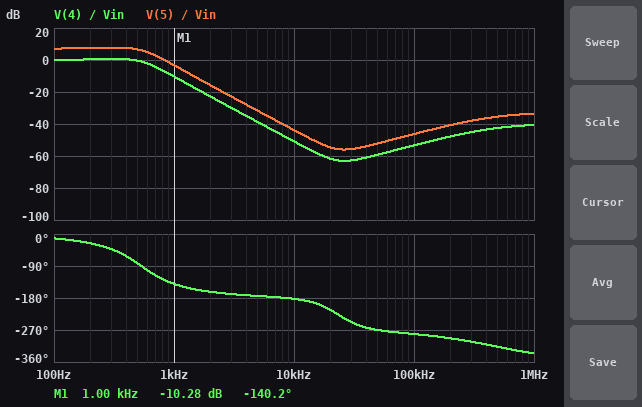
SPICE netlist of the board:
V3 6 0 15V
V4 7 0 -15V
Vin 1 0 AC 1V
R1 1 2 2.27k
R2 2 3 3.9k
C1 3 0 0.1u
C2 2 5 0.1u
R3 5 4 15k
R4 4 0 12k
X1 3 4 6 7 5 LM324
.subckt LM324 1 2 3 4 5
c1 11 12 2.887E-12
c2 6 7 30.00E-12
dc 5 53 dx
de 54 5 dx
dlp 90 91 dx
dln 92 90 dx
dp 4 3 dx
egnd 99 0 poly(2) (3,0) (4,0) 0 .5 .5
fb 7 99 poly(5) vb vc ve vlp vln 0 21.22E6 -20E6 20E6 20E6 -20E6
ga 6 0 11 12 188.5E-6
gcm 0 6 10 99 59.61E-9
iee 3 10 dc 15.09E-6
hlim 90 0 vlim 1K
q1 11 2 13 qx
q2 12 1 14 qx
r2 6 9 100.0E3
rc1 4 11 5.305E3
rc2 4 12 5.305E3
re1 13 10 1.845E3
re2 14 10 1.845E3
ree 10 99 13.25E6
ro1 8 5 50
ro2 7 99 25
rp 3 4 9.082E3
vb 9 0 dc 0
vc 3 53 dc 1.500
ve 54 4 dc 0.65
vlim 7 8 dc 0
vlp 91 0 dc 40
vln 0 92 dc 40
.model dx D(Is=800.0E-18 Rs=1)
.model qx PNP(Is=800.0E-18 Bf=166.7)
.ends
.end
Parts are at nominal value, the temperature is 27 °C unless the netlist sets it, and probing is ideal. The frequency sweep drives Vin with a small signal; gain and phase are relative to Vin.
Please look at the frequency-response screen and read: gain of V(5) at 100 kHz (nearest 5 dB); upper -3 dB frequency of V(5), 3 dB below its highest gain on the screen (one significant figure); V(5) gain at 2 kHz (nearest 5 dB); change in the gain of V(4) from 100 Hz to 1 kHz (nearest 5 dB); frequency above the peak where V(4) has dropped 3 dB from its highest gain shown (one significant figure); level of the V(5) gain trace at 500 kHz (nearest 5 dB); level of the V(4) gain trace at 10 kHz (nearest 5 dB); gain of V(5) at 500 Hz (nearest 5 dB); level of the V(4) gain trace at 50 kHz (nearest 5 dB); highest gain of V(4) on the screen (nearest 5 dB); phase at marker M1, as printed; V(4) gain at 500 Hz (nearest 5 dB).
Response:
-45 dB
600 Hz
-15 dB
-10 dB
600 Hz
-35 dB
-50 dB
5 dB
-60 dB
0 dB
-140.2 deg
0 dB
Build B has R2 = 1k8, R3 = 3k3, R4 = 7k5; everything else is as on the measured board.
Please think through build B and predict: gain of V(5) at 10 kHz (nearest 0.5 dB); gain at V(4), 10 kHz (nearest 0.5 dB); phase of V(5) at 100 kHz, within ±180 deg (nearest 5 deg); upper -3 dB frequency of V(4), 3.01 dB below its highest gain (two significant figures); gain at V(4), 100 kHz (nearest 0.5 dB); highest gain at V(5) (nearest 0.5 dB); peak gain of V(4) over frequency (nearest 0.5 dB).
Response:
-41.0 dB
-44.0 dB
85 deg
730 Hz
-53.0 dB
3.0 dB
0 dB
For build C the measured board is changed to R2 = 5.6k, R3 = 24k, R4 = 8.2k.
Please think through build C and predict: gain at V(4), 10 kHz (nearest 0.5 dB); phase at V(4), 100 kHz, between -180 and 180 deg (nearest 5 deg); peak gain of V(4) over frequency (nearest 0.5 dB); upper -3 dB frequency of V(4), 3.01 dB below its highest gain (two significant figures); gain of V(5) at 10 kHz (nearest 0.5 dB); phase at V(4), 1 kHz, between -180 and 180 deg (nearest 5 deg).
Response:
-54.0 dB
70 deg
9.5 dB
500 Hz
-42.0 dB
-170 deg
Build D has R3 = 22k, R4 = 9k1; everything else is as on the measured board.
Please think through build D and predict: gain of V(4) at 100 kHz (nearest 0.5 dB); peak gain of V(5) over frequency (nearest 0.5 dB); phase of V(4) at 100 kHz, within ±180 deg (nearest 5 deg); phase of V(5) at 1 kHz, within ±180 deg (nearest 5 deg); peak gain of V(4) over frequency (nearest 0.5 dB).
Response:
-53.5 dB
23.5 dB
70 deg
-170 deg
13.0 dB
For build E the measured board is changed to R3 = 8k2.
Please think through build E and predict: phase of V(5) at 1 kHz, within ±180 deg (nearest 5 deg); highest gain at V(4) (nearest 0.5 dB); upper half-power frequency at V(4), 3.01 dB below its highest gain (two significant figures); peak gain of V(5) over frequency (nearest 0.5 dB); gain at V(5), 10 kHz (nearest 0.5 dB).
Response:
-130 deg
0 dB
480 Hz
4.5 dB
-46.5 dB
